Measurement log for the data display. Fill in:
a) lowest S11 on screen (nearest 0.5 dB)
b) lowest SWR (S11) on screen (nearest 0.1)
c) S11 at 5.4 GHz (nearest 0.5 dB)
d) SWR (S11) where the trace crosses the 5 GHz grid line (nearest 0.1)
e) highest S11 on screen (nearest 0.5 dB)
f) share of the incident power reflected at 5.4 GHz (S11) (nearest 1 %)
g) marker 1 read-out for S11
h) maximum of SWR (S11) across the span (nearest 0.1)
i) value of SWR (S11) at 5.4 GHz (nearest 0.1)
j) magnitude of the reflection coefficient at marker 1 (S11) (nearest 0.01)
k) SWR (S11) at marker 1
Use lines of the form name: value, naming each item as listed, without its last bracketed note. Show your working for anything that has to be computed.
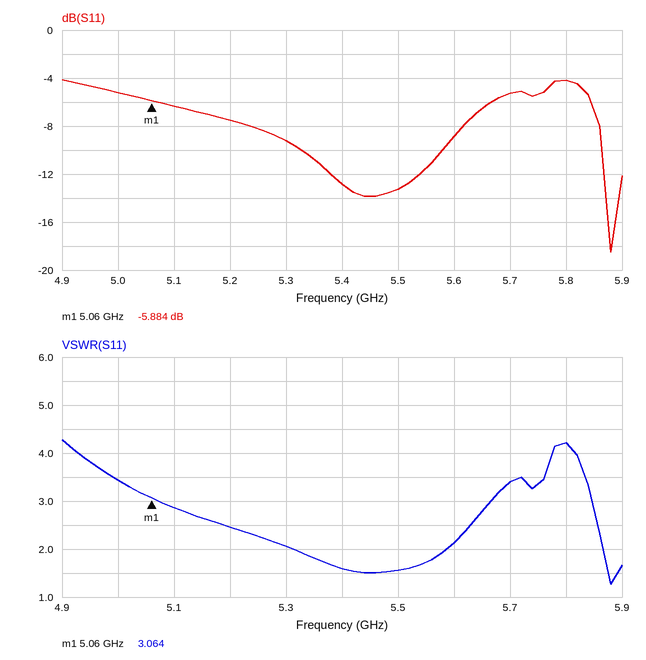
lowest S11 on screen: -18.5 dB
lowest SWR (S11) on screen: 1.3
S11 at 5.4 GHz: -13.0 dB
SWR (S11) where the trace crosses the 5 GHz grid line: 3.4
highest S11 on screen: -4.0 dB
share of the incident power reflected at 5.4 GHz (S11): 10^(-13/10) ≈ 5 %
marker 1 read-out for S11: -5.884 dB
maximum of SWR (S11) across the span: 4.3
value of SWR (S11) at 5.4 GHz: 1.6
magnitude of the reflection coefficient at marker 1 (S11): 10^(-5.884/20) ≈ 0.51
SWR (S11) at marker 1: 3.064
